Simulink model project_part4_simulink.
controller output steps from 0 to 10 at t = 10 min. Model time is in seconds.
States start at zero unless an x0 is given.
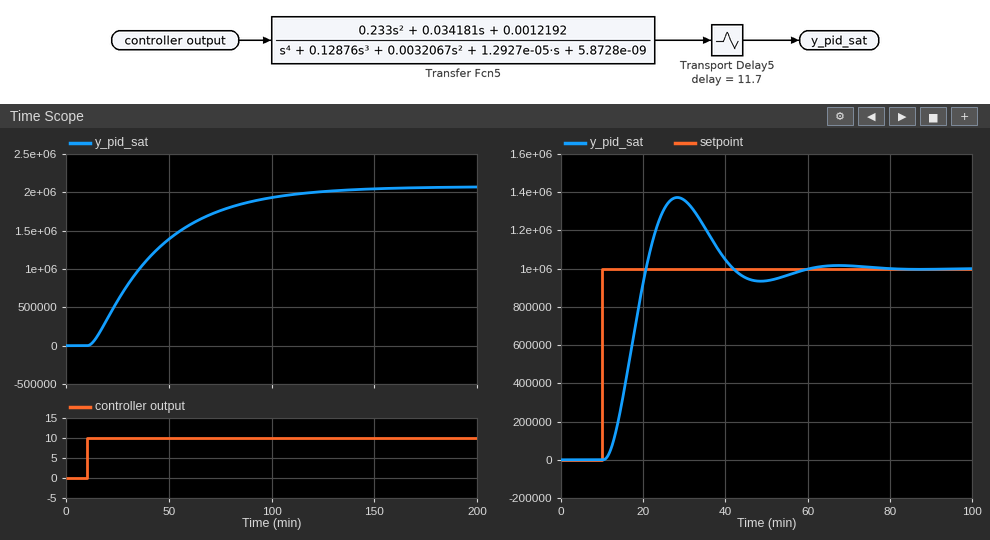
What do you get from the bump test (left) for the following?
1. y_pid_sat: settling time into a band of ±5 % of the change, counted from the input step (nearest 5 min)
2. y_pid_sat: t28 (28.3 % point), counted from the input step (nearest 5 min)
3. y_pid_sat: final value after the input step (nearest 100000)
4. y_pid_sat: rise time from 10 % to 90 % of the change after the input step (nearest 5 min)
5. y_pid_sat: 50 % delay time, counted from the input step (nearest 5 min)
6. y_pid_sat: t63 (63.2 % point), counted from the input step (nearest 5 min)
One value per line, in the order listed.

100 min
15 min
2100000
70 min
25 min
35 min
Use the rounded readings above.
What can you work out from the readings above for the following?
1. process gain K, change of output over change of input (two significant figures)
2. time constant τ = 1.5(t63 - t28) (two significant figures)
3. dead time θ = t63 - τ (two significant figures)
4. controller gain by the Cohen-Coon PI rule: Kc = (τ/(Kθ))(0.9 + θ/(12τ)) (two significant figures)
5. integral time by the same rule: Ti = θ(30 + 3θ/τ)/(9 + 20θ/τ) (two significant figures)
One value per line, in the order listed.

210000
30 min
5.0 min
0.000026
12 min
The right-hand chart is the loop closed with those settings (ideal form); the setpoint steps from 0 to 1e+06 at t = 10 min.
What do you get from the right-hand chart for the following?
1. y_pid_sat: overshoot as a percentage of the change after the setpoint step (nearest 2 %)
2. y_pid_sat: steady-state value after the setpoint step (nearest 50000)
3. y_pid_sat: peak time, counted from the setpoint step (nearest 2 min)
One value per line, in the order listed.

38 %
1000000
18 min
